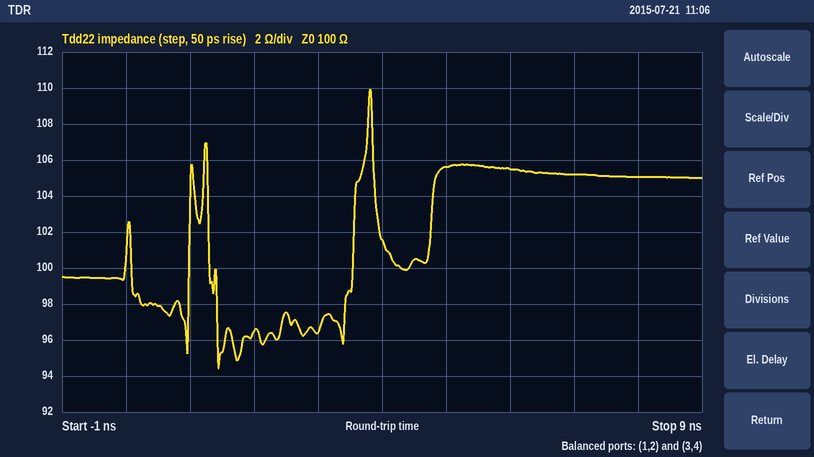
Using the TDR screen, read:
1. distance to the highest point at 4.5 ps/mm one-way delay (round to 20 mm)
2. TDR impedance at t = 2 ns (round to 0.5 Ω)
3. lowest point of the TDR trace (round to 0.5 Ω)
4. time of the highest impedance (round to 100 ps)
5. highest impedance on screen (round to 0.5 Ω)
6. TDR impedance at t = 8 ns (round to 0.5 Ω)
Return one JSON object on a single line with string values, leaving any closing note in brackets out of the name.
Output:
{"distance to the highest point at 4.5 ps/mm one-way delay": "420 mm", "TDR impedance at t = 2 ns": "96.5 Ω", "lowest point of the TDR trace": "94.5 Ω", "time of the highest impedance": "3.8 ns", "highest impedance on screen": "110.0 Ω", "TDR impedance at t = 8 ns": "105.0 Ω"}
